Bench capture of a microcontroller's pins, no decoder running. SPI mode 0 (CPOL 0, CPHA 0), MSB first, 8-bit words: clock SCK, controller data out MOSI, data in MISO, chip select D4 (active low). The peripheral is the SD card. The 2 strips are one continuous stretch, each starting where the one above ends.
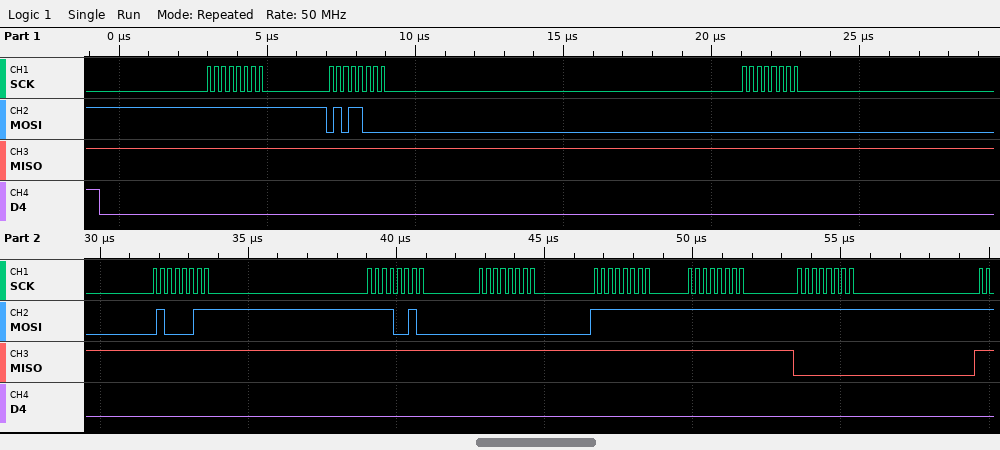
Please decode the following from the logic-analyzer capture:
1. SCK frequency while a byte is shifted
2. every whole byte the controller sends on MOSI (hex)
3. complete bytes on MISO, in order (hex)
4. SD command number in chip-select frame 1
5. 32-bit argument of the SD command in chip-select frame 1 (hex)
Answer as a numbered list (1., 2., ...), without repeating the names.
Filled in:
1. 4 MHz
2. 0xFF 0x58 0x00 0x43 0xF2 0x00 0xFF 0xFF 0xFF
3. 0xFF 0xFF 0xFF 0xFF 0xFF 0xFF 0xFF 0xFF 0x00
4. CMD24
5. 0x0043F200
